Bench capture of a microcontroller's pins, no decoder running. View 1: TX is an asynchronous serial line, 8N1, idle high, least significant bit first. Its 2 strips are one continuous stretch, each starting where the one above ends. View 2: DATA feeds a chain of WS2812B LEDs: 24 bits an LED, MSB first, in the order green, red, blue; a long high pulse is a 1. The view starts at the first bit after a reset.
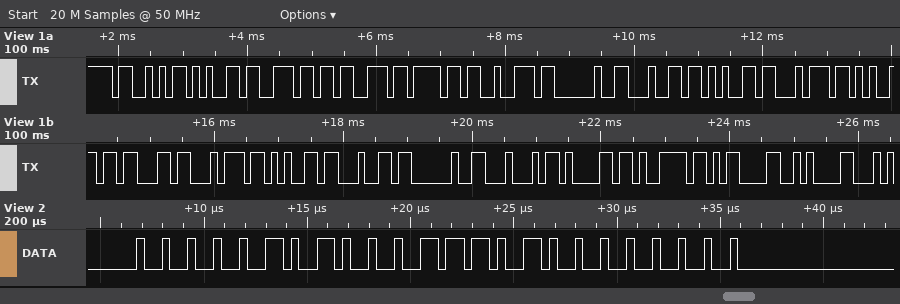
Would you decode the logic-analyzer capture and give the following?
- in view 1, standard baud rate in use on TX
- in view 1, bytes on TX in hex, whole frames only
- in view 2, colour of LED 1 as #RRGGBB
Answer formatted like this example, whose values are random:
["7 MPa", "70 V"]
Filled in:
["9600 baud", "0x53 0x65 0x6E 0x73 0x6F 0x72 0x20 0x64 0x65 0x74 0x65 0x63 0x74 0x65 0x64 0x20 0x44 0x61 0x79 0x0D 0x0A", "#1D0500"]
